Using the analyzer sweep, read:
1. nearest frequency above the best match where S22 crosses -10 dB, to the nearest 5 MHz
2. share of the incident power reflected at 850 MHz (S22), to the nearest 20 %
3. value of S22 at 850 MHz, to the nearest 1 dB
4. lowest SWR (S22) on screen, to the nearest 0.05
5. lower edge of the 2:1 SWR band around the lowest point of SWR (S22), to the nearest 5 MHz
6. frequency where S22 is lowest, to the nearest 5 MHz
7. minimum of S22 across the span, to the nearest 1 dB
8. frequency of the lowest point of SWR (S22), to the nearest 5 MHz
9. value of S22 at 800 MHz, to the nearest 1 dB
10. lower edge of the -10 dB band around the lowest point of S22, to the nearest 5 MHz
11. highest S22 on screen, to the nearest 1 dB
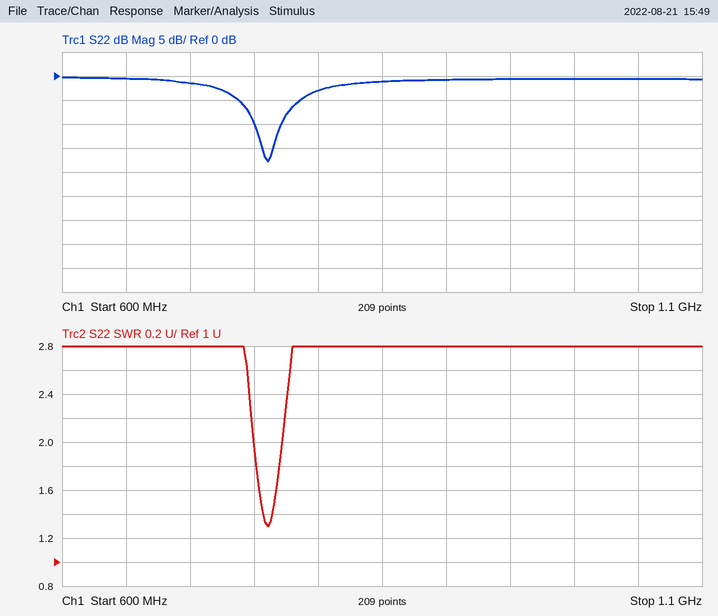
770 MHz
80 %
-1 dB
1.30
750 MHz
760 MHz
-18 dB
760 MHz
-3 dB
750 MHz
0 dB
